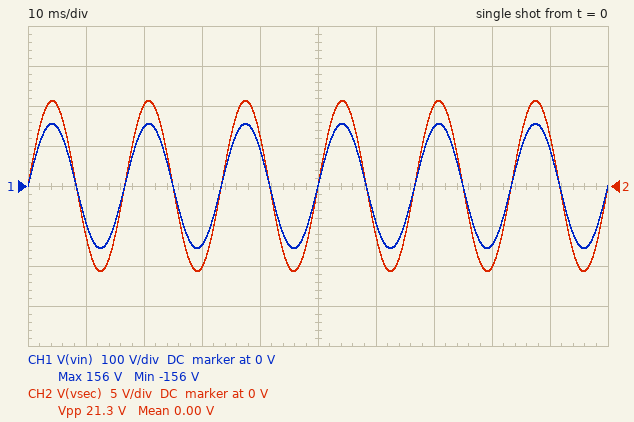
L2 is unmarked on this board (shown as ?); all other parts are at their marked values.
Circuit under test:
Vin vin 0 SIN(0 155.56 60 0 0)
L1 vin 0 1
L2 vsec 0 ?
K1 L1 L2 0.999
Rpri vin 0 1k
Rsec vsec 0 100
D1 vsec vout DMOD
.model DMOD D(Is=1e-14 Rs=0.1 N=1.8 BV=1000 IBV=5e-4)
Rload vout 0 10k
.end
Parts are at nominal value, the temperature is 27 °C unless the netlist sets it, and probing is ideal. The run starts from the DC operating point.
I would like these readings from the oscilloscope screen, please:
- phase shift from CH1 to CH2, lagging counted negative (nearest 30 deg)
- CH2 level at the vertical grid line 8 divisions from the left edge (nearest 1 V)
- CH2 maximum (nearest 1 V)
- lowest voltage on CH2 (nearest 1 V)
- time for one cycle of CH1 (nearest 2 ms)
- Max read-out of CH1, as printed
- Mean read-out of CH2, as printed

0 deg
-10 V
11 V
-11 V
16 ms
156 V
0.00 V
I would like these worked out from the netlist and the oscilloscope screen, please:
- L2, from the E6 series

4.7 mH
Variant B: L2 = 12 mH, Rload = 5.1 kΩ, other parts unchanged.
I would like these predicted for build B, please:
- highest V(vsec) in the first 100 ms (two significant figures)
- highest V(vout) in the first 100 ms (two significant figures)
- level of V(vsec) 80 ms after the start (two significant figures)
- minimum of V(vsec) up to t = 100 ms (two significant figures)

17 V
16 V
-16 V
-17 V
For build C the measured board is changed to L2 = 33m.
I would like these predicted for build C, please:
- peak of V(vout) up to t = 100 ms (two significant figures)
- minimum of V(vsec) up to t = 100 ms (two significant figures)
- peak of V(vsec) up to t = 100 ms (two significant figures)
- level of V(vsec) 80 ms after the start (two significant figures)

27 V
-28 V
28 V
-27 V
